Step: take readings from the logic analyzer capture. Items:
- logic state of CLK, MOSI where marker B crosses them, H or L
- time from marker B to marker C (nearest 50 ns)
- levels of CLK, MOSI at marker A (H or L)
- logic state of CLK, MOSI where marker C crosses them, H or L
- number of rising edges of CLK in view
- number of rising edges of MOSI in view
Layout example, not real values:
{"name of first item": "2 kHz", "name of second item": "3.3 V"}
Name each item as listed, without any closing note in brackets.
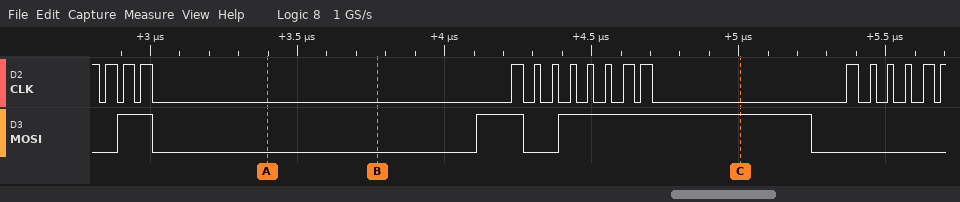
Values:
{"logic state of CLK, MOSI where marker B crosses them, H or L": "CLK=L, MOSI=L", "time from marker B to marker C": "1250 ns", "levels of CLK, MOSI at marker A": "CLK=L, MOSI=L", "logic state of CLK, MOSI where marker C crosses them, H or L": "CLK=L, MOSI=H", "number of rising edges of CLK in view": "17", "number of rising edges of MOSI in view": "3"}
